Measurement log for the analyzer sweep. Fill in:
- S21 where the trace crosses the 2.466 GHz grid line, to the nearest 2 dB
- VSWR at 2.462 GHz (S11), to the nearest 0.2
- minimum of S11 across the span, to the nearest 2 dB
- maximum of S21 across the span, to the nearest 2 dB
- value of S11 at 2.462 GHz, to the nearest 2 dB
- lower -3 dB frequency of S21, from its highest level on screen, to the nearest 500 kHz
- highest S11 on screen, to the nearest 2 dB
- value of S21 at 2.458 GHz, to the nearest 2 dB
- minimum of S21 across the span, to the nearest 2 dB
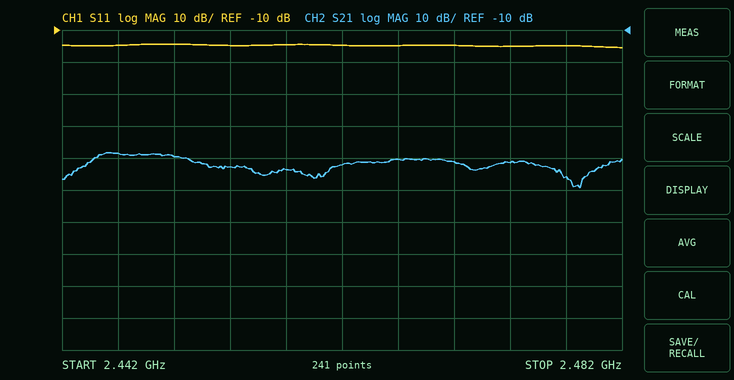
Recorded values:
-50 dB
1.4
-16 dB
-48 dB
-14 dB
2.4440 GHz
-14 dB
-54 dB
-60 dB
